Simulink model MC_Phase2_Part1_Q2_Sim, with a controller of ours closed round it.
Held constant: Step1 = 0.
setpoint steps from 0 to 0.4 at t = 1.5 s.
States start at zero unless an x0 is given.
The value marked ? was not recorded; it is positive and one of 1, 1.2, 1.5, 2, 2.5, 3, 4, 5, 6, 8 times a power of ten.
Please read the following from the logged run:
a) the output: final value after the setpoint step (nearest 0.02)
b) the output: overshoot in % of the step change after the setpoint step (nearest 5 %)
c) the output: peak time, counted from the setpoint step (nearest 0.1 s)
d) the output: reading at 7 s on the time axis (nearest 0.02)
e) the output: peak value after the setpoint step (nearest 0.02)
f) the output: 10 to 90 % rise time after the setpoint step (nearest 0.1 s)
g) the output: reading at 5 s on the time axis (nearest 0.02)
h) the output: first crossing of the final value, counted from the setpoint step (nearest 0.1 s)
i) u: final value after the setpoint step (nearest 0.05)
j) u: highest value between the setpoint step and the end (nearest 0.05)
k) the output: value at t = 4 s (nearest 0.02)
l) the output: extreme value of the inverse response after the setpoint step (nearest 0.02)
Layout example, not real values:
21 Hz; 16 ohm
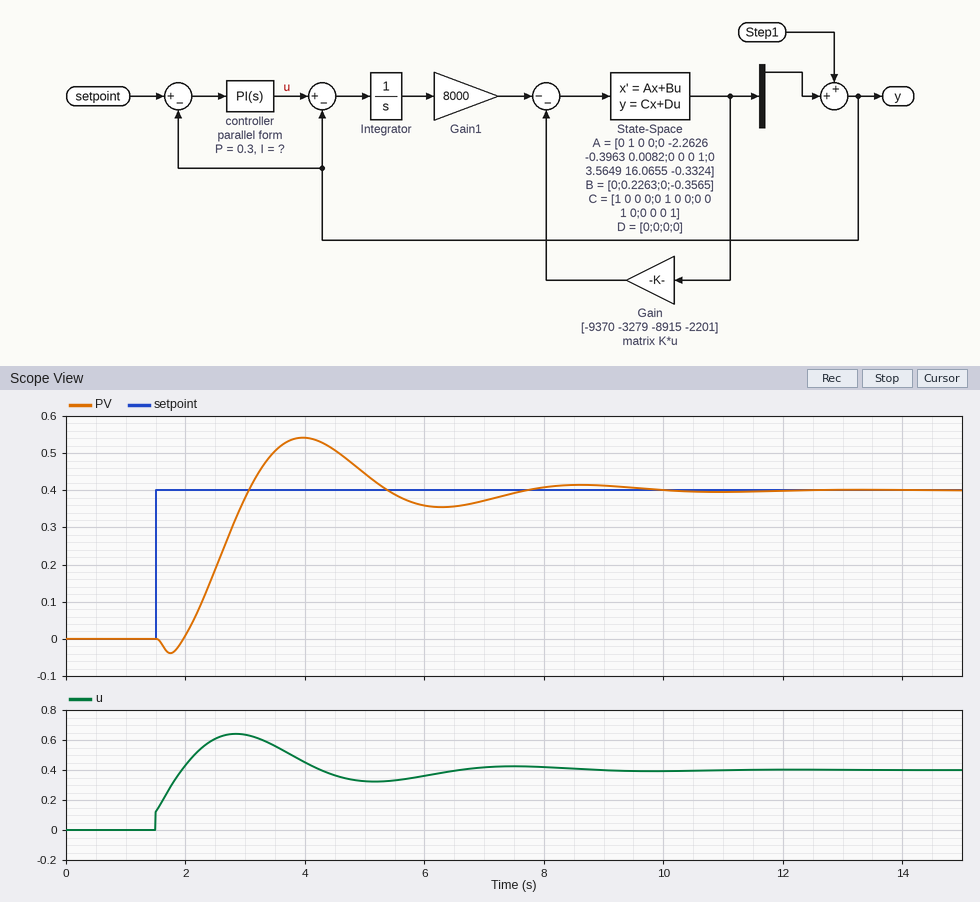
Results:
0.40; 35 %; 2.5 s; 0.38; 0.54; 0.8 s; 0.44; 1.6 s; 0.40; 0.65; 0.54; -0.04
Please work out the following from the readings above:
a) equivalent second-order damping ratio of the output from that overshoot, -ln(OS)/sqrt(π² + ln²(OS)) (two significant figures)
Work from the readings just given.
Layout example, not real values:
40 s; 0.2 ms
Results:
0.32
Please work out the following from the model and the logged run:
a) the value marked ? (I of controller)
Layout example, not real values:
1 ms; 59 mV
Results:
1.5
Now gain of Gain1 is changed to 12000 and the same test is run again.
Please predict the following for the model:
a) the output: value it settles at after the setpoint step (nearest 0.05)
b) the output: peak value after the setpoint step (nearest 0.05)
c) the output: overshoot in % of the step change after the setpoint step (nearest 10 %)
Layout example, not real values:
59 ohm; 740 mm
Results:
0.40; 0.50; 20 %
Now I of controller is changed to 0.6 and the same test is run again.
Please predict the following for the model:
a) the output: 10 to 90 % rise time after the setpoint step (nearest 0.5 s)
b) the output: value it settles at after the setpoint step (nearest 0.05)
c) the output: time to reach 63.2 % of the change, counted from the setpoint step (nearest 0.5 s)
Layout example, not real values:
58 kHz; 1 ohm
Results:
2.5 s; 0.40; 2.0 s
